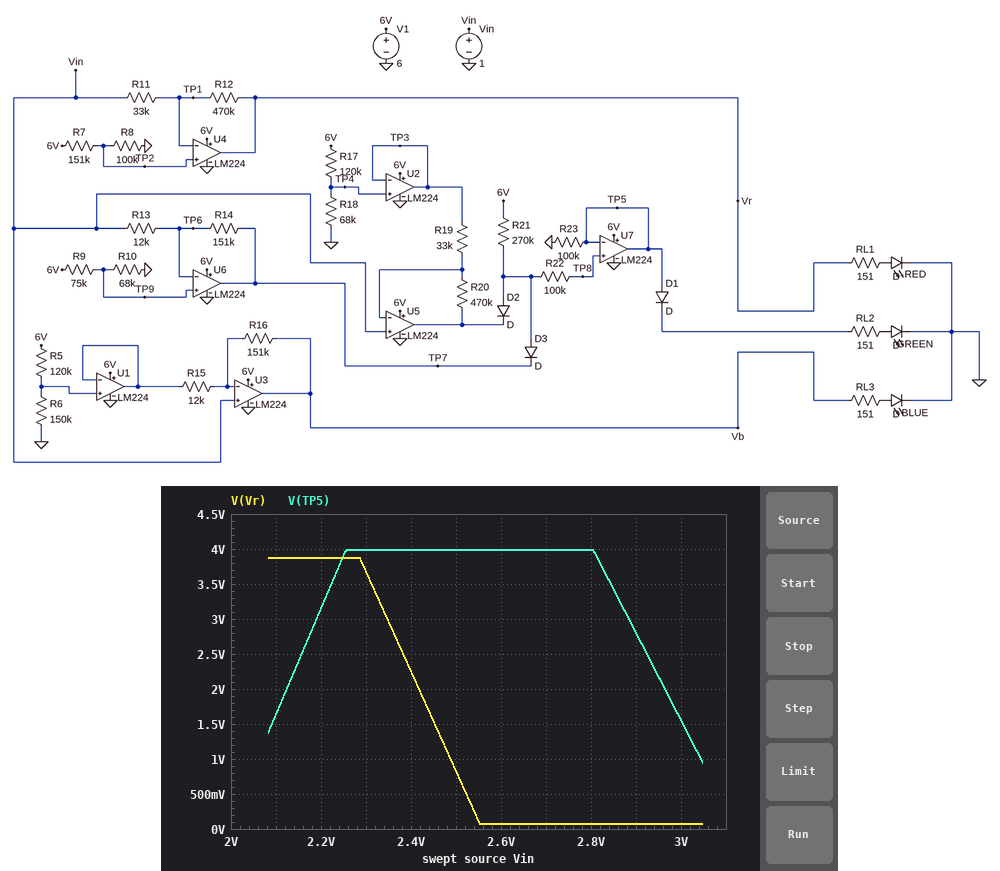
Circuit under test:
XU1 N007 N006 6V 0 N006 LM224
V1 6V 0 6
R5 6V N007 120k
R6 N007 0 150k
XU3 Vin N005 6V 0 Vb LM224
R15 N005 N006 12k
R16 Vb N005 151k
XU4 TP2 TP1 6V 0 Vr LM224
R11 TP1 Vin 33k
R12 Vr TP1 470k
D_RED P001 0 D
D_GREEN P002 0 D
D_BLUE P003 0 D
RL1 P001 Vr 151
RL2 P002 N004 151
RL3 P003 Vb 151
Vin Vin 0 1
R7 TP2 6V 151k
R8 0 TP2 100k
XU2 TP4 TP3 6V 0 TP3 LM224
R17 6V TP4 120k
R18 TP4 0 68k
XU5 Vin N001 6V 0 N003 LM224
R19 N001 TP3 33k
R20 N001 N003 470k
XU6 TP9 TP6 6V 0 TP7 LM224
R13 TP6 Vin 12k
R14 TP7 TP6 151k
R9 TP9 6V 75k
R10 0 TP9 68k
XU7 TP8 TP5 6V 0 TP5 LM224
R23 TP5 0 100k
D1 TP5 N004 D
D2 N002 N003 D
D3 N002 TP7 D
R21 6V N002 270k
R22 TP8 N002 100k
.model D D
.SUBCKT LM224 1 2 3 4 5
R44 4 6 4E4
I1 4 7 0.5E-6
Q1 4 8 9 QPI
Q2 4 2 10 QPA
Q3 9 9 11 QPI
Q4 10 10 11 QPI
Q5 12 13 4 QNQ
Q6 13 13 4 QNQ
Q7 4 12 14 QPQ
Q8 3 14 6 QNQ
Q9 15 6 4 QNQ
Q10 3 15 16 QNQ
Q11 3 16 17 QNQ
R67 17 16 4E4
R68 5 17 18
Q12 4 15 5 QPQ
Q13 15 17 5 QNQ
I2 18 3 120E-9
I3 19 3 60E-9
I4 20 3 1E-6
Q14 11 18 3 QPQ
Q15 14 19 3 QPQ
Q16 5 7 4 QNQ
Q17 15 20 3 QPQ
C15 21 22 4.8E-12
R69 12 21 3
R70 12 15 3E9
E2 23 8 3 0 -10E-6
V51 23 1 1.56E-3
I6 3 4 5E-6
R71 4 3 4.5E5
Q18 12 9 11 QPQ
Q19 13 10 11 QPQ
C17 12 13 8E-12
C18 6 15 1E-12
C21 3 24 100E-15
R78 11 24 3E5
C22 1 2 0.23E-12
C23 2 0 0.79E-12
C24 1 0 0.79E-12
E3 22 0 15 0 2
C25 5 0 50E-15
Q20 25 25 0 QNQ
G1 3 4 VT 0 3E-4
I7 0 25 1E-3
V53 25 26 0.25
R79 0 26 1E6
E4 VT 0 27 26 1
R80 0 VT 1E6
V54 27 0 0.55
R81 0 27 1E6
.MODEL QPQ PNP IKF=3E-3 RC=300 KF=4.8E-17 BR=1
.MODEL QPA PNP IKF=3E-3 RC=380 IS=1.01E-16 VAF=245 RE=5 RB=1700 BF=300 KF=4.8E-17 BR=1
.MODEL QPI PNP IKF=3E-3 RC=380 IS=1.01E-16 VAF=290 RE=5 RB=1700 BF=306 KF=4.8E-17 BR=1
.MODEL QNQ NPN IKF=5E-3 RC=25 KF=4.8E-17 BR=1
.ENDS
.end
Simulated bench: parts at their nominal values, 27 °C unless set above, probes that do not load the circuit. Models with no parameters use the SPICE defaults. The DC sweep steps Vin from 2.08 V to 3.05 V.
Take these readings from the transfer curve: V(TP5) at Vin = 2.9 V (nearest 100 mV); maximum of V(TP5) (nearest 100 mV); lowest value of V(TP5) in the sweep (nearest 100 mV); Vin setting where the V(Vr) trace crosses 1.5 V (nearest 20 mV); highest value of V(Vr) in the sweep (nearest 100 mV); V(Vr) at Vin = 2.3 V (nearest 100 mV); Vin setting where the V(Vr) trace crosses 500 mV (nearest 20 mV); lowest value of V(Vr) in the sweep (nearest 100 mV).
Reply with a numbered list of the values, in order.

1. 2.8 V
2. 4.0 V
3. 900 mV
4. 2.46 V
5. 3.9 V
6. 3.7 V
7. 2.52 V
8. 100 mV
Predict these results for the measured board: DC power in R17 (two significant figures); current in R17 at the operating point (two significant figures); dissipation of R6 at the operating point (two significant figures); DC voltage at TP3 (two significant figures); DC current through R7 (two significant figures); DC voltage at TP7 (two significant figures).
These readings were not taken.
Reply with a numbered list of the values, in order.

1. 120 µW
2. 32 µA
3. 74 µW
4. 2.2 V
5. 24 µA
6. 4.6 V
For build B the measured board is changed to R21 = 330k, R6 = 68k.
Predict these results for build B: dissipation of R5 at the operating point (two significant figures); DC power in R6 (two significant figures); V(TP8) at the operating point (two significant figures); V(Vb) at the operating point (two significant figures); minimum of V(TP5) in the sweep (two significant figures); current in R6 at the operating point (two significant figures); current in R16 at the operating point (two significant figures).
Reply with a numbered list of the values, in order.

1. 120 µW
2. 69 µW
3. 660 mV
4. 94 mV
5. 920 mV
6. 32 µA
7. 13 µA
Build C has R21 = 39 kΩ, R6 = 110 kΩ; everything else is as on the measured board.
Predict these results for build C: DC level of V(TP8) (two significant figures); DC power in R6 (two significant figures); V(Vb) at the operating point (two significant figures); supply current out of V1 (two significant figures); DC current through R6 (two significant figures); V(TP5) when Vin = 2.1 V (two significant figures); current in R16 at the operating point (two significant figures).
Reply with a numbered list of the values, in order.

1. 1.3 V
2. 75 µW
3. 100 mV
4. 24 mA
5. 26 µA
6. 1.7 V
7. 17 µA
